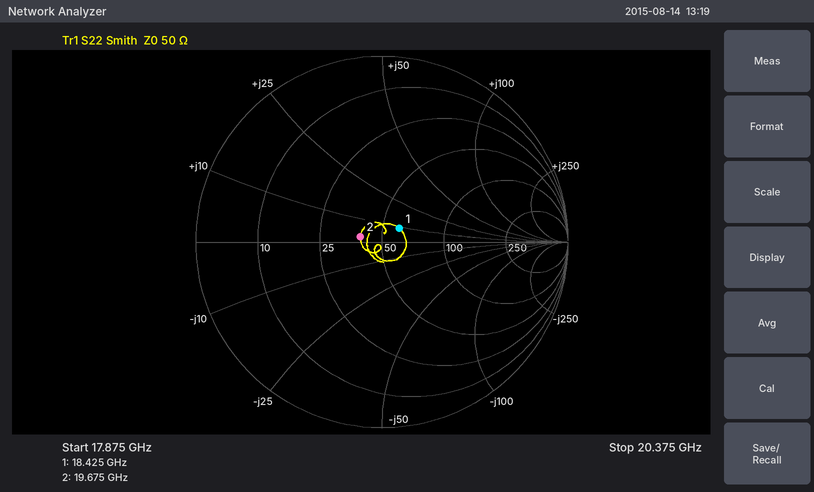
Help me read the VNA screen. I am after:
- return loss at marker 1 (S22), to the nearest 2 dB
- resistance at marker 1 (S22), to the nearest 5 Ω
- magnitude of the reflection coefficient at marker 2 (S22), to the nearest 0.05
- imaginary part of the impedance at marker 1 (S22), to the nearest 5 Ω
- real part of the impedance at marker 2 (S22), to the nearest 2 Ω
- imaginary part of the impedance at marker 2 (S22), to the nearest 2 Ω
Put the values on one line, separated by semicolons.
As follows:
18 dB; 60 Ω; 0.10; +10 Ω; 40 Ω; +2 Ω
